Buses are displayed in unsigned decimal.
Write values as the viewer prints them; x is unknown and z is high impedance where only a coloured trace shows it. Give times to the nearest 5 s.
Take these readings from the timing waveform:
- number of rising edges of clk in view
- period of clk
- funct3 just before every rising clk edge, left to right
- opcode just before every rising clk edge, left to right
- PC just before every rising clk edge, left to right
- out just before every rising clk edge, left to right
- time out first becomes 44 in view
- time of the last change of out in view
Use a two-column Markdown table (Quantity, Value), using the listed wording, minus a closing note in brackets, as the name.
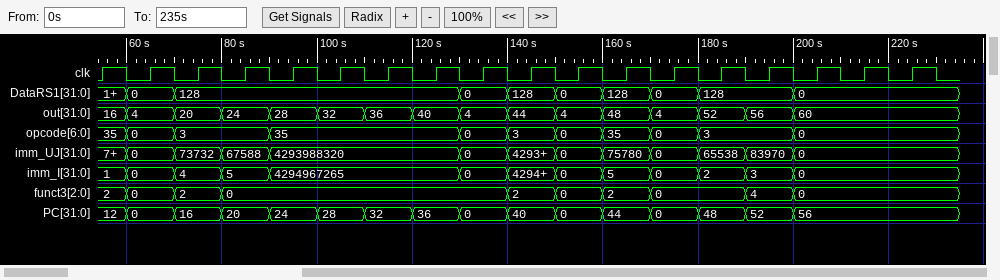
| Quantity | Value |
|---|---|
| number of rising edges of clk in view | 18 |
| period of clk | 10 s |
| funct3 just before every rising clk edge, left to right | 2, 0, 2, 0, 0, 0, 0, 0, 0, 2, 0, 2, 0, 0, 4, 0, 0, 0 |
| opcode just before every rising clk edge, left to right | 35, 0, 3, 3, 35, 35, 35, 35, 0, 3, 0, 35, 0, 3, 3, 0, 0, 0 |
| PC just before every rising clk edge, left to right | 12, 0, 16, 20, 24, 28, 32, 36, 0, 40, 0, 44, 0, 48, 52, 56, 56, 56 |
| out just before every rising clk edge, left to right | 16, 4, 20, 24, 28, 32, 36, 40, 4, 44, 4, 48, 4, 52, 56, 60, 60, 60 |
| time out first becomes 44 in view | 140 s |
| time of the last change of out in view | 200 s |
